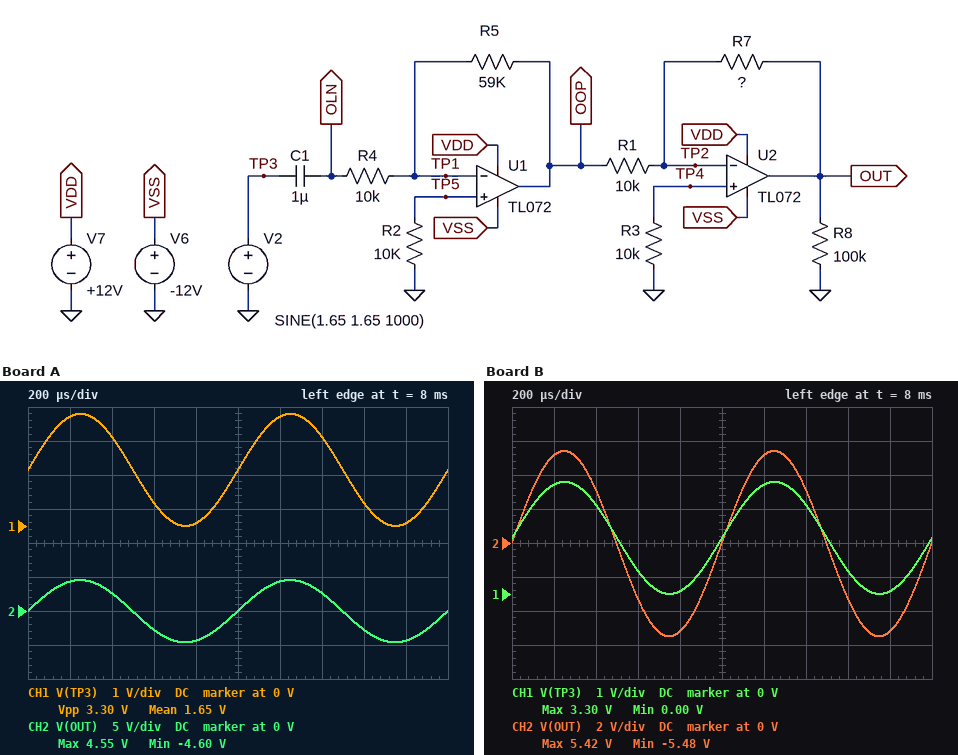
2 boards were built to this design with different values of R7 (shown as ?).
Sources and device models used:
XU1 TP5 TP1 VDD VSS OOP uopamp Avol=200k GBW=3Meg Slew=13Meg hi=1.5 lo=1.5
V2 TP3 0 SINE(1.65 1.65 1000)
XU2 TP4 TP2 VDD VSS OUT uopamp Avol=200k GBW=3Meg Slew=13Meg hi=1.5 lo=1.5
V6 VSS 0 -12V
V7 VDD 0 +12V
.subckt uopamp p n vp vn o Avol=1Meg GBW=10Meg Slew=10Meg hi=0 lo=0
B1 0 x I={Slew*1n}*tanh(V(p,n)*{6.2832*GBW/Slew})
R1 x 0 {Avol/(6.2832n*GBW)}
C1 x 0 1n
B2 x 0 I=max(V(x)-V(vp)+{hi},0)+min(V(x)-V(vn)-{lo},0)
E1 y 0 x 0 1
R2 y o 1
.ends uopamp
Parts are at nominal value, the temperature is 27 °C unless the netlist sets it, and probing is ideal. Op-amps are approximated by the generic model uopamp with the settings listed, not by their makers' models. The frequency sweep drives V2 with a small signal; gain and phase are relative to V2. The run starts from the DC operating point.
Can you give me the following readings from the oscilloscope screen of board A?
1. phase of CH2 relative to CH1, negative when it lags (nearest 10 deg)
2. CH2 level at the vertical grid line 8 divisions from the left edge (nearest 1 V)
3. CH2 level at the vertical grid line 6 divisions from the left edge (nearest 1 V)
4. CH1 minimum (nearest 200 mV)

0 deg
-3 V
4 V
0 V
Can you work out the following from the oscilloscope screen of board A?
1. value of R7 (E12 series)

4.7 kΩ
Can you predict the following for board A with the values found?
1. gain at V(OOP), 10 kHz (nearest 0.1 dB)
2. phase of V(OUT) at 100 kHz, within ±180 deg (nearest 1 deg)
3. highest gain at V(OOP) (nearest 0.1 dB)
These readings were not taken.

15.4 dB
-16 deg
15.4 dB
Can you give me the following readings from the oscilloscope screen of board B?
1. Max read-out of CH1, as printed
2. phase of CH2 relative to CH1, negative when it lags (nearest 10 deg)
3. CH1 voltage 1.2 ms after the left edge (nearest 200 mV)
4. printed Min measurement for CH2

3.30 V
0 deg
3.2 V
-5.48 V
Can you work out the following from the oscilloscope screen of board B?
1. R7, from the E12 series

5.6 kΩ
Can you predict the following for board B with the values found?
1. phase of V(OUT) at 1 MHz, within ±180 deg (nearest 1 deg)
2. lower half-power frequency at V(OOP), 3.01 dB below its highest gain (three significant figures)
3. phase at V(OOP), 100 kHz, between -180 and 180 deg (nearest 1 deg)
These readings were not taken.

-94 deg
15.9 Hz
167 deg
